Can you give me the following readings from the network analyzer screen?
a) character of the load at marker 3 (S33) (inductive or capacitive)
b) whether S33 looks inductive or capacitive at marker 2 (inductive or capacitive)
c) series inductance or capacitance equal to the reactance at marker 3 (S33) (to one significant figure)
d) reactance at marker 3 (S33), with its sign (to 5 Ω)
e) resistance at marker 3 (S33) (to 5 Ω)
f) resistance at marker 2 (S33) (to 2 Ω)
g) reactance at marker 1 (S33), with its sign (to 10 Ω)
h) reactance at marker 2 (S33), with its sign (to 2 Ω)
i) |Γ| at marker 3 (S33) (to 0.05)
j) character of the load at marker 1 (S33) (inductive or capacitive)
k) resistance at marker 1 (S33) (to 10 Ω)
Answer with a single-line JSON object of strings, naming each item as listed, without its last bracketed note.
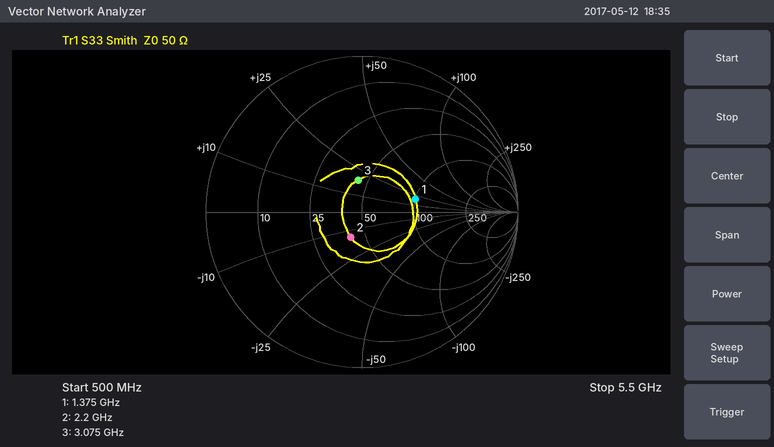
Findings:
{"character of the load at marker 3 (S33)": "inductive", "whether S33 looks inductive or capacitive at marker 2": "capacitive", "series inductance or capacitance equal to the reactance at marker 3 (S33)": "1.0 nH", "reactance at marker 3 (S33), with its sign": "+20 Ω", "resistance at marker 3 (S33)": "45 Ω", "resistance at marker 2 (S33)": "42 Ω", "reactance at marker 1 (S33), with its sign": "+20 Ω", "reactance at marker 2 (S33), with its sign": "-14 Ω", "|Γ| at marker 3 (S33)": "0.20", "character of the load at marker 1 (S33)": "inductive", "resistance at marker 1 (S33)": "100 Ω"}
